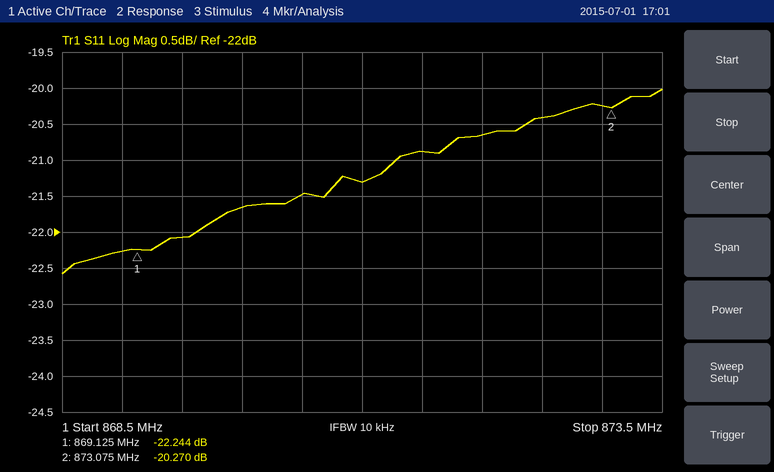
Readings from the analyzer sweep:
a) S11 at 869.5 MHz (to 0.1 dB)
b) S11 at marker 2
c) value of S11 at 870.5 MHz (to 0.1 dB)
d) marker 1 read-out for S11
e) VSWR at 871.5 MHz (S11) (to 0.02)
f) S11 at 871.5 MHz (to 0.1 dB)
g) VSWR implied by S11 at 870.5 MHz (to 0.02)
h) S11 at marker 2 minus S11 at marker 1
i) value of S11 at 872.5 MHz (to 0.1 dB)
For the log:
-22.1 dB
-20.270 dB
-21.5 dB
-22.244 dB
1.20
-20.9 dB
1.18
1.974 dB
-20.4 dB
